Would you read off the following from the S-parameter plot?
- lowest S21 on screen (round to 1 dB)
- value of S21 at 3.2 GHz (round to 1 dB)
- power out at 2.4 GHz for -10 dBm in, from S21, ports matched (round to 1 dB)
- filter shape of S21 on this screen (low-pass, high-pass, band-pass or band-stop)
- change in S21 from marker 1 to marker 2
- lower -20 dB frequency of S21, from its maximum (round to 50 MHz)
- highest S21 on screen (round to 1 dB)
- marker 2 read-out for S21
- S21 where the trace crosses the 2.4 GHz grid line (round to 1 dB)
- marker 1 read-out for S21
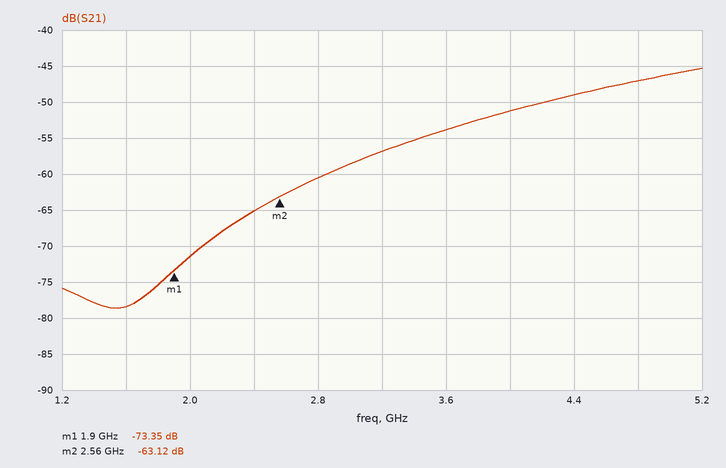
-79 dB
-57 dB
-75 dBm
high-pass
10.23 dB
2.40 GHz
-45 dB
-63.12 dB
-65 dB
-73.35 dB
